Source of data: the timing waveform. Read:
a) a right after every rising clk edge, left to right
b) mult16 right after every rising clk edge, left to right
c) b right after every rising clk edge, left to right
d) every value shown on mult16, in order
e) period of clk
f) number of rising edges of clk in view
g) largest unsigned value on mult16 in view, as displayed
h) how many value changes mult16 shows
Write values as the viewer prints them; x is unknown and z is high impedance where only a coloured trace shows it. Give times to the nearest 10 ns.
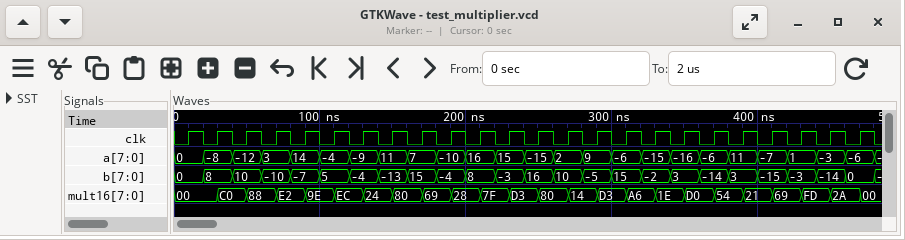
0, -8, -12, 3, 14, -4, -9, 11, 7, -10, 16, 15, -15, 2, 9, -6, -15, -16, -6, 11, -7, 1, -3, -6
00, C0, 88, E2, 9E, EC, 24, 80, 69, 28, 7F, D3, 80, 14, D3, A6, 1E, D0, 54, 21, 69, FD, 2A, 00
0, 8, 10, -10, -7, 5, -4, -13, 15, -4, 8, -3, 16, 10, -5, 15, -2, 3, -14, 3, -15, -3, -14, 0
00, C0, 88, E2, 9E, EC, 24, 80, 69, 28, 7F, D3, 80, 14, D3, A6, 1E, D0, 54, 21, 69, FD, 2A, 00
20 ns
24
FD
23
